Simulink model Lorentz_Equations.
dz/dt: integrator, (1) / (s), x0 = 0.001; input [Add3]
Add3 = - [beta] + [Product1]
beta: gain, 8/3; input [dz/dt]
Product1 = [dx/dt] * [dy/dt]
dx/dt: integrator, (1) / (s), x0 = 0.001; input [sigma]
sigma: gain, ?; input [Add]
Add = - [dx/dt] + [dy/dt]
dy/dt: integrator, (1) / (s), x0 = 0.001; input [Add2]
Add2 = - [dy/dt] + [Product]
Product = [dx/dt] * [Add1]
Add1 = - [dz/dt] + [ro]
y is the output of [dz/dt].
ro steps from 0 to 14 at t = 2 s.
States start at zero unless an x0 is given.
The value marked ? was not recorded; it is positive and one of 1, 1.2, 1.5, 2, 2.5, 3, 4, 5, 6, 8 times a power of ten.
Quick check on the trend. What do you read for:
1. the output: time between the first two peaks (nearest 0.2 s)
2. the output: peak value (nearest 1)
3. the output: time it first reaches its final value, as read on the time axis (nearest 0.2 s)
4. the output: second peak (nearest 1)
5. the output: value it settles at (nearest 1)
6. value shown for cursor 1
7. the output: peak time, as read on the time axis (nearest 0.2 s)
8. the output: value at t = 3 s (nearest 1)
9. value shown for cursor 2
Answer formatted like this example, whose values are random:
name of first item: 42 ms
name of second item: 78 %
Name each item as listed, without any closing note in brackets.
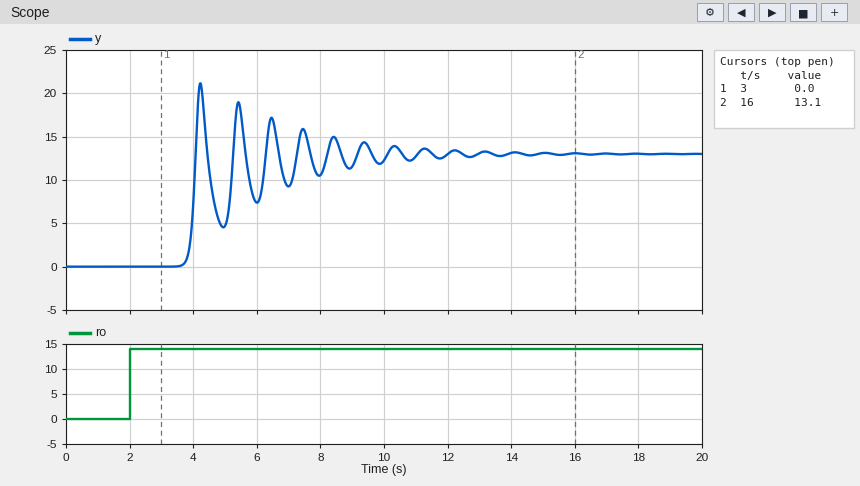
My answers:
the output: time between the first two peaks: 1.2 s
the output: peak value: 21
the output: time it first reaches its final value, as read on the time axis: 4.0 s
the output: second peak: 19
the output: value it settles at: 13
value shown for cursor 1: 0.0
the output: peak time, as read on the time axis: 4.2 s
the output: value at t = 3 s: 0
value shown for cursor 2: 13.1
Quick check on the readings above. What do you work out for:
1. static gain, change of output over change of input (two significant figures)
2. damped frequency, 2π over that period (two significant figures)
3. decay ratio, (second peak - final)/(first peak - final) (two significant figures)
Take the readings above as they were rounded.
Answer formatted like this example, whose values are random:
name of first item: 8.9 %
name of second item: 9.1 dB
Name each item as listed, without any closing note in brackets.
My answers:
static gain, change of output over change of input: 0.93
damped frequency, 2π over that period: 5.2 rad/s
decay ratio, (second peak - final)/(first peak - final): 0.75
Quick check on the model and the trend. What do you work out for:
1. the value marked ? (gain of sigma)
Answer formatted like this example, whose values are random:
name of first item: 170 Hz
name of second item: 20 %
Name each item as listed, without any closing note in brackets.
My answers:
the value marked ?: 5
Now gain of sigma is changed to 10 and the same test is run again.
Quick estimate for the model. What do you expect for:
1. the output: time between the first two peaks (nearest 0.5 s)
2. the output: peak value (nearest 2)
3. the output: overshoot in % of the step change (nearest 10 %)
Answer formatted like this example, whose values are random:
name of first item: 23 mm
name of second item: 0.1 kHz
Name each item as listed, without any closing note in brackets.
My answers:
the output: time between the first two peaks: 1.5 s
the output: peak value: 22
the output: overshoot in % of the step change: 70 %
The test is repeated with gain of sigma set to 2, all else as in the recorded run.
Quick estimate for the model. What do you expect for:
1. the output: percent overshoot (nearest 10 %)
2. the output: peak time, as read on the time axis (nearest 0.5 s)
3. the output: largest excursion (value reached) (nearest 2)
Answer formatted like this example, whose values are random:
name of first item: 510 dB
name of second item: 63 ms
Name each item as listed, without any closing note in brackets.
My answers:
the output: percent overshoot: 50 %
the output: peak time, as read on the time axis: 5.0 s
the output: largest excursion (value reached): 20
